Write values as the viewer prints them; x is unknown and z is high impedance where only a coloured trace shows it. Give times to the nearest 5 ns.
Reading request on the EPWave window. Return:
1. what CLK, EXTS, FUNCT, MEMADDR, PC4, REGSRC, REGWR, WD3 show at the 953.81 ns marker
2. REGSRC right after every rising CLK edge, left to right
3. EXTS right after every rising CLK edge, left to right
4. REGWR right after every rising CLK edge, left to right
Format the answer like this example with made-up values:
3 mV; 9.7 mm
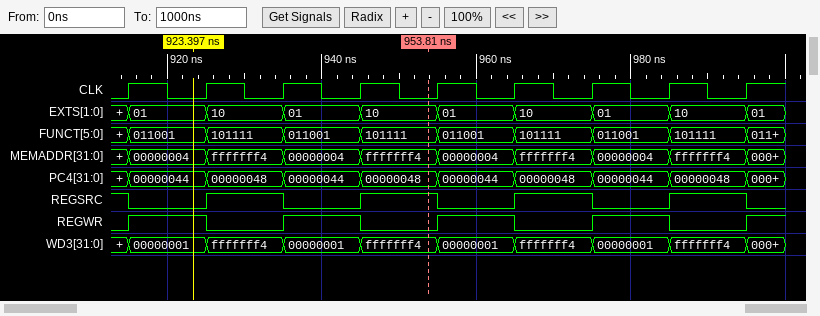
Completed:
CLK=0, EXTS=10, FUNCT=101111, MEMADDR=fffffff4, PC4=00000048, REGSRC=1, REGWR=0, WD3=fffffff4; 0 1 0 1 0 1 0 1 0; 01, 10, 01, 10, 01, 10, 01, 10, 01; 1 0 1 0 1 0 1 0 1
